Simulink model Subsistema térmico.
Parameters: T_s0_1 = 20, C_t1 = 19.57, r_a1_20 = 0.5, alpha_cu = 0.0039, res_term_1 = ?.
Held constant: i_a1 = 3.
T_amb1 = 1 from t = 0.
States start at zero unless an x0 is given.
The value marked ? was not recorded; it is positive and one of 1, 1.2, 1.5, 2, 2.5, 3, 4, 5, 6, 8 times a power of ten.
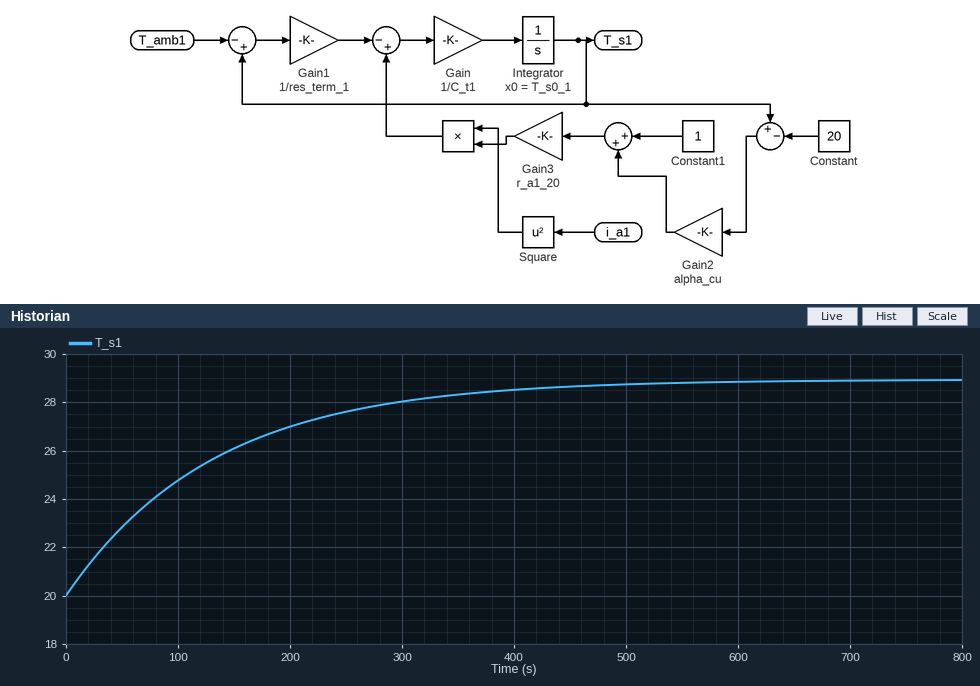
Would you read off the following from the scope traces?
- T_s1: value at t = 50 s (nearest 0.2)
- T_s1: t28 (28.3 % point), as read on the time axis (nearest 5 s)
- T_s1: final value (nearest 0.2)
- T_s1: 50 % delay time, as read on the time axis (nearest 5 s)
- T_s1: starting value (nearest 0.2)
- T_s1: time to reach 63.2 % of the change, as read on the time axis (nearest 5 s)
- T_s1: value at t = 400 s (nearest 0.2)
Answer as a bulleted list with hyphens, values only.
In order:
- 22.8
- 45 s
- 29.0
- 90 s
- 20.0
- 130 s
- 28.6
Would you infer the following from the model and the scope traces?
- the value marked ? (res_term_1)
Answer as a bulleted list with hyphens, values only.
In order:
- 6
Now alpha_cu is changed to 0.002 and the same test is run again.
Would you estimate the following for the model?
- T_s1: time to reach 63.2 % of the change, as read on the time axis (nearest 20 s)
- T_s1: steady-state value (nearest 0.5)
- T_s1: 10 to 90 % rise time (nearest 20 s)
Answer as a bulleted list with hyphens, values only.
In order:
- 120 s
- 28.5
- 280 s
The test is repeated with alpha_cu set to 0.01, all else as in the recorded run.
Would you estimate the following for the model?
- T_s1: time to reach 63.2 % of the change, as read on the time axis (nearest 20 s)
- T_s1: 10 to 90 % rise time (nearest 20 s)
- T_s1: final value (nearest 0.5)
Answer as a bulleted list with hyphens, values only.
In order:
- 160 s
- 360 s
- 31.0
